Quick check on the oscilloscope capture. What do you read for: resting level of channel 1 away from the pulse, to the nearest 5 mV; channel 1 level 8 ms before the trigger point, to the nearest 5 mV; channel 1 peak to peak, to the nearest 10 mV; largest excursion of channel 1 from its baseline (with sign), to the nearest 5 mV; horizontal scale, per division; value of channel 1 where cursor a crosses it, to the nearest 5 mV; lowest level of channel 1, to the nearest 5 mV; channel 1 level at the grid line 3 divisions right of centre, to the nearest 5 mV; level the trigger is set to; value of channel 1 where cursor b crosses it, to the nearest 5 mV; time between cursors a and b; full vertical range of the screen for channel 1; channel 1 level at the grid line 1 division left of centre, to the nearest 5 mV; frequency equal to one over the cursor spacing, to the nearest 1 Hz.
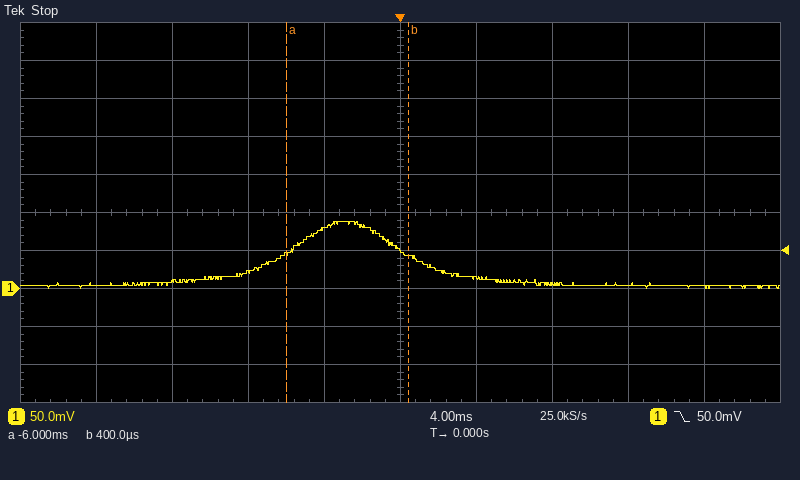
5 mV
20 mV
90 mV
+85 mV
4 ms
45 mV
0 mV
5 mV
50.0 mV
45 mV
6.4 ms
500 mV
80 mV
156 Hz
